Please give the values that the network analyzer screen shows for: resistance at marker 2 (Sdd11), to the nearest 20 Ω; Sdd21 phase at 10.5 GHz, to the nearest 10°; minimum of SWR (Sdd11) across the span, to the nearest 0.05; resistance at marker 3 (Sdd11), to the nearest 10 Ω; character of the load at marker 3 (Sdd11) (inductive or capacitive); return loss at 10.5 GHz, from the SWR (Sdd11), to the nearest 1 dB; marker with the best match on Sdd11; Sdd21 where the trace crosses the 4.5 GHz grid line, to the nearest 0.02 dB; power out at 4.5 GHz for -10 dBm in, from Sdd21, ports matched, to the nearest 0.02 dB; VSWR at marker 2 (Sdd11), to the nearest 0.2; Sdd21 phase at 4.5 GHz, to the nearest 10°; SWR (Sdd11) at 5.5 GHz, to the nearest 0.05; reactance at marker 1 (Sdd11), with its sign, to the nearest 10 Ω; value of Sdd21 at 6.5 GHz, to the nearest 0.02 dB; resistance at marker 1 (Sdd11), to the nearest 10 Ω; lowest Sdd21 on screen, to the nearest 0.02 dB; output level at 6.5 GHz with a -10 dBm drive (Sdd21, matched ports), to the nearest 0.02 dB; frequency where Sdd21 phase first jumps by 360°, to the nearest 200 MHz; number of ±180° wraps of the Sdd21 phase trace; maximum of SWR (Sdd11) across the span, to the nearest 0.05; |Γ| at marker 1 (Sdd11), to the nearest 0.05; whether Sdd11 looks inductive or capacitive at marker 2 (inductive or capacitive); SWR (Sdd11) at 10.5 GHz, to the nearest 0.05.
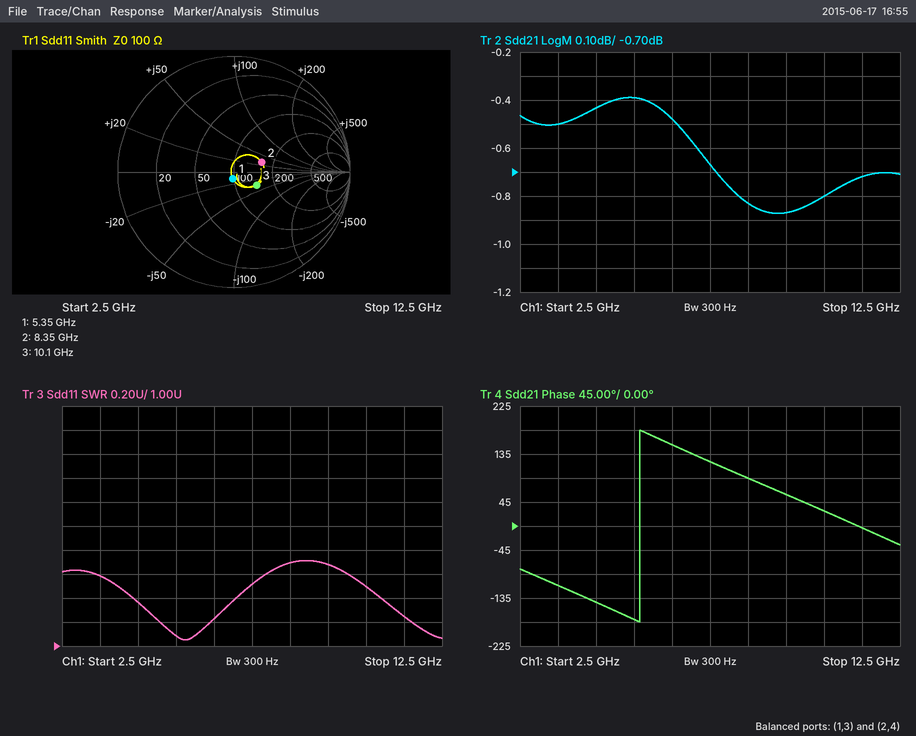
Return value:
160 Ω
30°
1.05
140 Ω
capacitive
14 dB
marker 1
-0.44 dB
-10.44 dBm
1.6
-140°
1.10
-10 Ω
-0.48 dB
100 Ω
-0.88 dB
-10.48 dBm
5.6 GHz
1
1.70
0.05
inductive
1.50
